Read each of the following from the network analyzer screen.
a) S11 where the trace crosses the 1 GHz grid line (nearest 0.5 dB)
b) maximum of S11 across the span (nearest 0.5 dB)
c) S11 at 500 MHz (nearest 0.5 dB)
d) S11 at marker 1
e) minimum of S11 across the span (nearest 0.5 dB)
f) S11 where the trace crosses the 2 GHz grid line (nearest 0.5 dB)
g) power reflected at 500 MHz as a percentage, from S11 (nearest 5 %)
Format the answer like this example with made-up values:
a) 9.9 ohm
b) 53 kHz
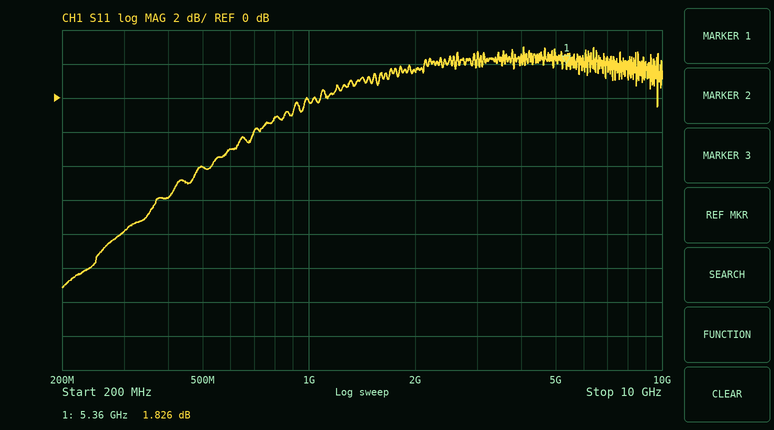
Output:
a) 0.0 dB
b) 3.0 dB
c) -4.0 dB
d) 1.826 dB
e) -11.0 dB
f) 1.5 dB
g) 40 %
